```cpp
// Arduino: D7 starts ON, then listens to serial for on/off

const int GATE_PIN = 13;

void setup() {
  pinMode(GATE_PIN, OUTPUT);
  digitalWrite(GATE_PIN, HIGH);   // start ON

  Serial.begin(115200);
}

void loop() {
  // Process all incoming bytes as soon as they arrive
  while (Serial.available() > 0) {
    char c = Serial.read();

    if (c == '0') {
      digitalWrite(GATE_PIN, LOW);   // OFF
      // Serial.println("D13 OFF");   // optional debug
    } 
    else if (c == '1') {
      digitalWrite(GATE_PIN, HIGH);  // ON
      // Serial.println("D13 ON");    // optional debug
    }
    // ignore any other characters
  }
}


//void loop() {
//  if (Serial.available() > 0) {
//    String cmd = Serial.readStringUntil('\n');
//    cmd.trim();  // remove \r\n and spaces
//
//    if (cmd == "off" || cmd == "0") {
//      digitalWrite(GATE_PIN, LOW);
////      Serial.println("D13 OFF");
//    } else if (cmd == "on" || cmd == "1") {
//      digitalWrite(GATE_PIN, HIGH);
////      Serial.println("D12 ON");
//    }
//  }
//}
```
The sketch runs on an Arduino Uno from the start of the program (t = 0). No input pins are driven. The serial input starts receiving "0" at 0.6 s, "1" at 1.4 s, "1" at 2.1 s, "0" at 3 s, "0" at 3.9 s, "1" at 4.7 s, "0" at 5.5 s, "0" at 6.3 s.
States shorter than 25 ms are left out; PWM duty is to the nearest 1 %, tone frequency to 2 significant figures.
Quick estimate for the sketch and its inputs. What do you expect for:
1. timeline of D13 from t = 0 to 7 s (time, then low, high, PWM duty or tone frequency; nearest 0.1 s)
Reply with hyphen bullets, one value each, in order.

- 0 s high; 0.6 s low; 1.4 s high; 3 s low; 4.7 s high; 5.5 s low
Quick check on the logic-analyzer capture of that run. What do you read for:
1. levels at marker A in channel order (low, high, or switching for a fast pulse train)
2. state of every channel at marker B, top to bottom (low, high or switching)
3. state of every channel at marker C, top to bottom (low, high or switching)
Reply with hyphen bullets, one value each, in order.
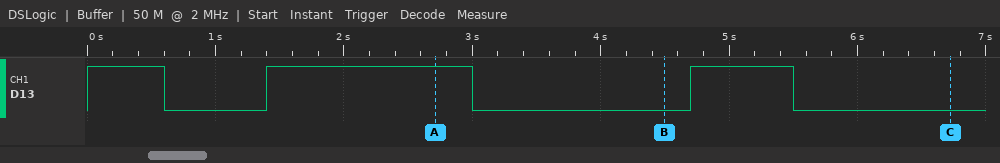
- D13 high
- D13 low
- D13 low
